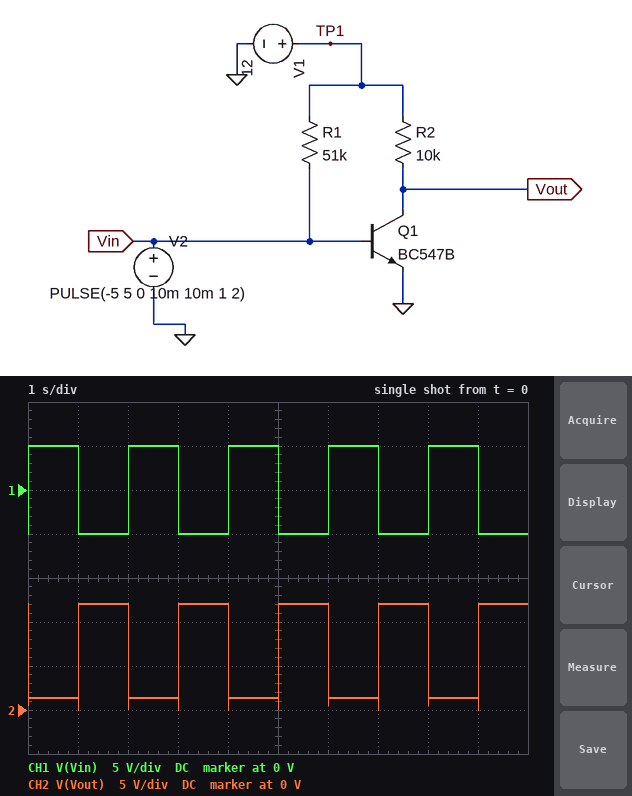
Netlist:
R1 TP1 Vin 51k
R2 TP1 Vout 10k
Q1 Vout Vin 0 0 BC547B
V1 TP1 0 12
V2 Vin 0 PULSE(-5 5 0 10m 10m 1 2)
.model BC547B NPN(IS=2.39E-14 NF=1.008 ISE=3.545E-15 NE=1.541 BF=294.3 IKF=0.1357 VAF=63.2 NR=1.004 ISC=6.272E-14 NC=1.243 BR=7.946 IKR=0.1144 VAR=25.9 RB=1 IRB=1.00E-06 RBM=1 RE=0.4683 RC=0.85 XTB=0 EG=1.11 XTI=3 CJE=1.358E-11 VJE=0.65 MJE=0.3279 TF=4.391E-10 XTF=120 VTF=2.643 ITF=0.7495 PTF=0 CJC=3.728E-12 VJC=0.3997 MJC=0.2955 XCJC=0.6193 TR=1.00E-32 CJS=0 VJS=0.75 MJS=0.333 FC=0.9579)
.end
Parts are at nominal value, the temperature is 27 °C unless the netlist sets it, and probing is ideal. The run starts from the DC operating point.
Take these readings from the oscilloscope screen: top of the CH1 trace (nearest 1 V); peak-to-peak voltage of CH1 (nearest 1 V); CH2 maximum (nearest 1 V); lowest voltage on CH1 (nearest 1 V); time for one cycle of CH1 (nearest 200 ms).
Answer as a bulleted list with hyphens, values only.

- 5 V
- 10 V
- 12 V
- -5 V
- 2.0 s
